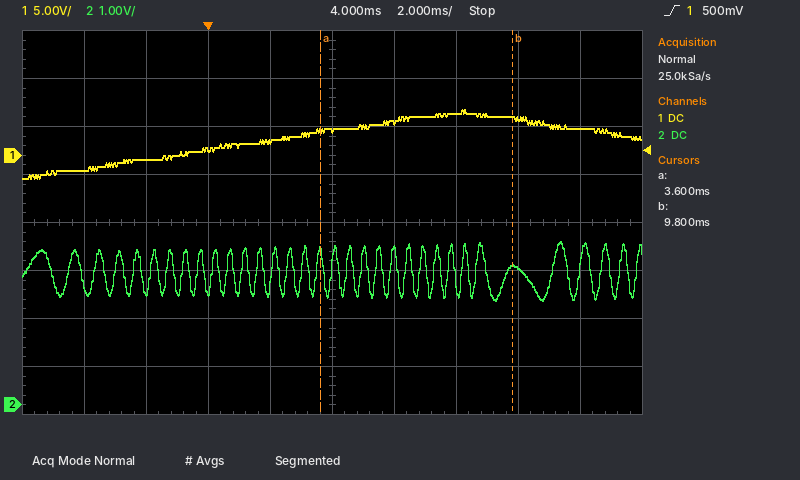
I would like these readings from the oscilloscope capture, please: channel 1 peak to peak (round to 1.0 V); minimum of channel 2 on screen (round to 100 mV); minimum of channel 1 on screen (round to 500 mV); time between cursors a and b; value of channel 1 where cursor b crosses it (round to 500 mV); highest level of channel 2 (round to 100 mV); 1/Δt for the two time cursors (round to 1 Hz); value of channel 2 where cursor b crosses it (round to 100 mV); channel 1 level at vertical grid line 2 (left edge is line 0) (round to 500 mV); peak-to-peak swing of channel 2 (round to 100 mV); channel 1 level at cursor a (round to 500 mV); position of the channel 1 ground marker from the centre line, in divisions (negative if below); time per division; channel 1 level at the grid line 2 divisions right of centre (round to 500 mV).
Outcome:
7.0 V
2.2 V
-2.5 V
6.2 ms
4.0 V
3.4 V
161 Hz
2.9 V
-500 mV
1.2 V
2.5 V
+1.4 div
2 ms
4.5 V
